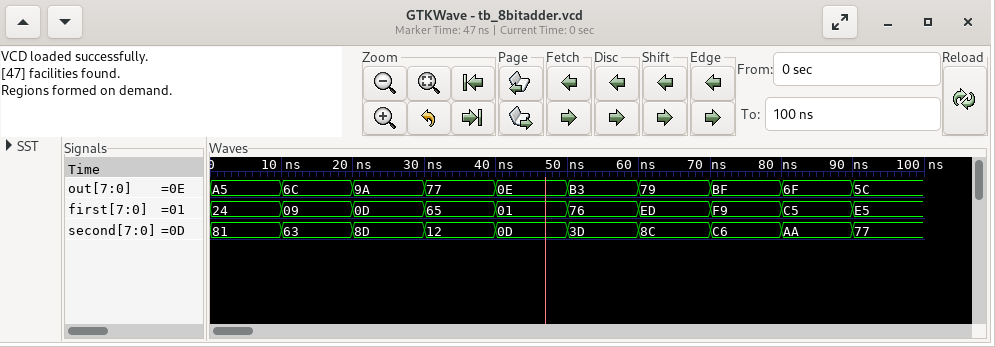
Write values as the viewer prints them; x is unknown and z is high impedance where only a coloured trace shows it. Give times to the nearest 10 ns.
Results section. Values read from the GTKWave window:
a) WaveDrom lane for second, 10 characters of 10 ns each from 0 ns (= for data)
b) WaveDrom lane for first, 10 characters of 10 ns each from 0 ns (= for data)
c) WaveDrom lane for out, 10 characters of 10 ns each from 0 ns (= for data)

{name: 'second', wave: '==========', data: '81 63 8D 12 0D 3D 8C C6 AA 77'}
{name: 'first', wave: '==========', data: '24 09 0D 65 01 76 ED F9 C5 E5'}
{name: 'out', wave: '==========', data: 'A5 6C 9A 77 0E B3 79 BF 6F 5C'}
